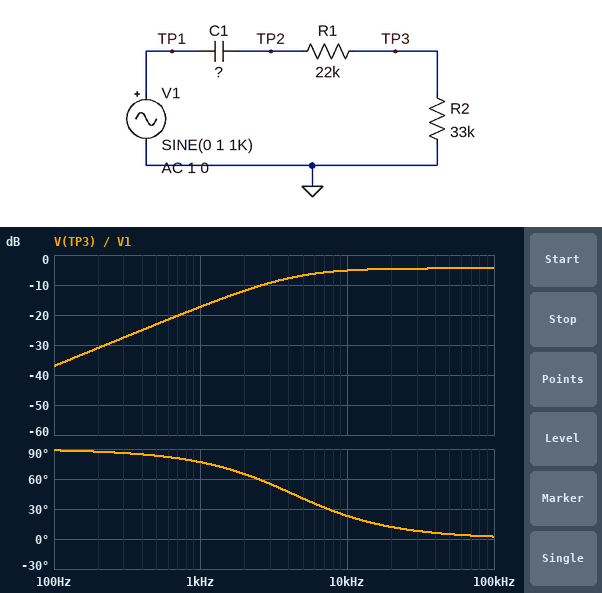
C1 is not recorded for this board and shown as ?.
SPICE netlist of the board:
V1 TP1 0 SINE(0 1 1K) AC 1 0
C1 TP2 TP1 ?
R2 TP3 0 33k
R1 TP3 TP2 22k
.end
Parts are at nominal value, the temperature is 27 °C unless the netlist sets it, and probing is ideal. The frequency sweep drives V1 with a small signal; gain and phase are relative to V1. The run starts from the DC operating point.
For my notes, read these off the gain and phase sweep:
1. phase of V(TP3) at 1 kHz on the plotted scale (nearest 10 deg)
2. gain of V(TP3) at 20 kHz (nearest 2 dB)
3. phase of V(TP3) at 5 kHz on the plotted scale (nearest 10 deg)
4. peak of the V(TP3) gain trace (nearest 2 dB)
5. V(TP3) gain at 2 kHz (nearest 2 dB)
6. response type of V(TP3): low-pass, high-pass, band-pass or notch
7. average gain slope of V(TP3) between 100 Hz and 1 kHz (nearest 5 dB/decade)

80 deg
-4 dB
40 deg
-4 dB
-12 dB
high-pass
20 dB/decade
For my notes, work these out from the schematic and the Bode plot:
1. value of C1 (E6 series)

680 pF
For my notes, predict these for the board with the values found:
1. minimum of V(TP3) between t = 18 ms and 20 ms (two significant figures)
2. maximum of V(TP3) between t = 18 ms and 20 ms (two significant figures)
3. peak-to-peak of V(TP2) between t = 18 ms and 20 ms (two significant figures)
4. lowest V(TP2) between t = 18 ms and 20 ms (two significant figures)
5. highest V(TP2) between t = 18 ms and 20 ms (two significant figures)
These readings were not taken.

-140 mV
140 mV
460 mV
-230 mV
230 mV
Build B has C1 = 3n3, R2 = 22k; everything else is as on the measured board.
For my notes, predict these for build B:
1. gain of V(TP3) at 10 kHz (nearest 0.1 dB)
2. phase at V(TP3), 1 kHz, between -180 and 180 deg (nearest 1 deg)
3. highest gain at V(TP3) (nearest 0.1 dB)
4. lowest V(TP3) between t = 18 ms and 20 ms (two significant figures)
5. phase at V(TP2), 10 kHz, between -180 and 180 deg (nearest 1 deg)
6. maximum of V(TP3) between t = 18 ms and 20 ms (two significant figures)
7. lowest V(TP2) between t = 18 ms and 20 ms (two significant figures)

-6.1 dB
48 deg
-6.0 dB
-340 mV
6 deg
340 mV
-670 mV
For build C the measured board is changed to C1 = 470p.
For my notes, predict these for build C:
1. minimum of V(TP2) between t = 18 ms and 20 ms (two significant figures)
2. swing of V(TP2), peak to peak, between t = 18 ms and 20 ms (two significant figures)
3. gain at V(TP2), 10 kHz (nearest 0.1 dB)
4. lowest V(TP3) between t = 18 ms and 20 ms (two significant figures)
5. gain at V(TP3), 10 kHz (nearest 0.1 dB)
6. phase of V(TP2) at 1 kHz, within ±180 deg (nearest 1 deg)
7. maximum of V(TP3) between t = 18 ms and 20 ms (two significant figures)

-160 mV
320 mV
-1.4 dB
-96 mV
-5.8 dB
81 deg
96 mV
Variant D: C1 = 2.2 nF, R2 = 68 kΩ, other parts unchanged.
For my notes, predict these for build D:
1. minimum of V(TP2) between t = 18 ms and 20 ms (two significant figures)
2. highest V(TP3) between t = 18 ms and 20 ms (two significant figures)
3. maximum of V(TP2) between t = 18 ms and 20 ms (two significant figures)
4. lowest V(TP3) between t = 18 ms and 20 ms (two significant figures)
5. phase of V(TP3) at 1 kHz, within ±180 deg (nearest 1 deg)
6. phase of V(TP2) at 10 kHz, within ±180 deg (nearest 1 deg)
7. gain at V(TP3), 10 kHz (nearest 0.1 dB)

-780 mV
590 mV
780 mV
-590 mV
39 deg
5 deg
-2.5 dB
